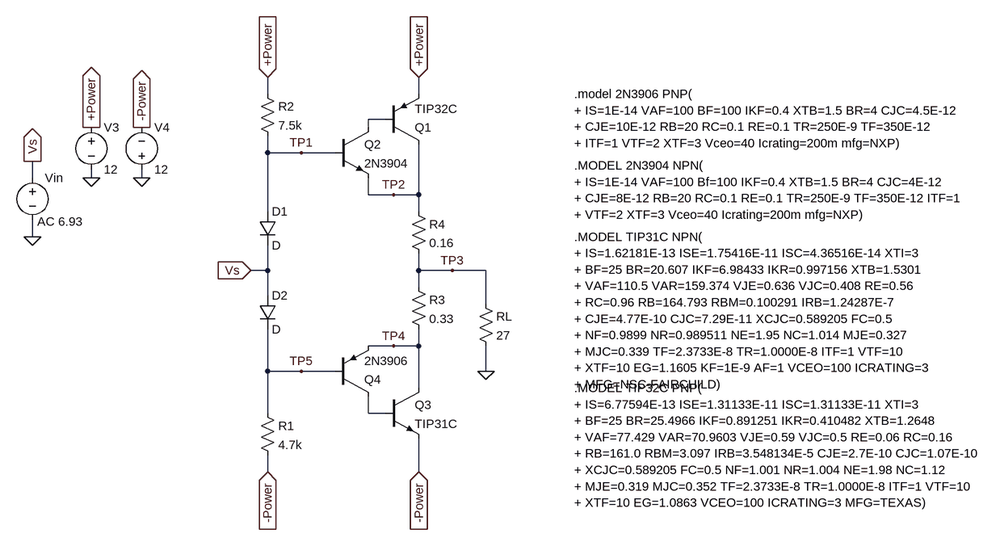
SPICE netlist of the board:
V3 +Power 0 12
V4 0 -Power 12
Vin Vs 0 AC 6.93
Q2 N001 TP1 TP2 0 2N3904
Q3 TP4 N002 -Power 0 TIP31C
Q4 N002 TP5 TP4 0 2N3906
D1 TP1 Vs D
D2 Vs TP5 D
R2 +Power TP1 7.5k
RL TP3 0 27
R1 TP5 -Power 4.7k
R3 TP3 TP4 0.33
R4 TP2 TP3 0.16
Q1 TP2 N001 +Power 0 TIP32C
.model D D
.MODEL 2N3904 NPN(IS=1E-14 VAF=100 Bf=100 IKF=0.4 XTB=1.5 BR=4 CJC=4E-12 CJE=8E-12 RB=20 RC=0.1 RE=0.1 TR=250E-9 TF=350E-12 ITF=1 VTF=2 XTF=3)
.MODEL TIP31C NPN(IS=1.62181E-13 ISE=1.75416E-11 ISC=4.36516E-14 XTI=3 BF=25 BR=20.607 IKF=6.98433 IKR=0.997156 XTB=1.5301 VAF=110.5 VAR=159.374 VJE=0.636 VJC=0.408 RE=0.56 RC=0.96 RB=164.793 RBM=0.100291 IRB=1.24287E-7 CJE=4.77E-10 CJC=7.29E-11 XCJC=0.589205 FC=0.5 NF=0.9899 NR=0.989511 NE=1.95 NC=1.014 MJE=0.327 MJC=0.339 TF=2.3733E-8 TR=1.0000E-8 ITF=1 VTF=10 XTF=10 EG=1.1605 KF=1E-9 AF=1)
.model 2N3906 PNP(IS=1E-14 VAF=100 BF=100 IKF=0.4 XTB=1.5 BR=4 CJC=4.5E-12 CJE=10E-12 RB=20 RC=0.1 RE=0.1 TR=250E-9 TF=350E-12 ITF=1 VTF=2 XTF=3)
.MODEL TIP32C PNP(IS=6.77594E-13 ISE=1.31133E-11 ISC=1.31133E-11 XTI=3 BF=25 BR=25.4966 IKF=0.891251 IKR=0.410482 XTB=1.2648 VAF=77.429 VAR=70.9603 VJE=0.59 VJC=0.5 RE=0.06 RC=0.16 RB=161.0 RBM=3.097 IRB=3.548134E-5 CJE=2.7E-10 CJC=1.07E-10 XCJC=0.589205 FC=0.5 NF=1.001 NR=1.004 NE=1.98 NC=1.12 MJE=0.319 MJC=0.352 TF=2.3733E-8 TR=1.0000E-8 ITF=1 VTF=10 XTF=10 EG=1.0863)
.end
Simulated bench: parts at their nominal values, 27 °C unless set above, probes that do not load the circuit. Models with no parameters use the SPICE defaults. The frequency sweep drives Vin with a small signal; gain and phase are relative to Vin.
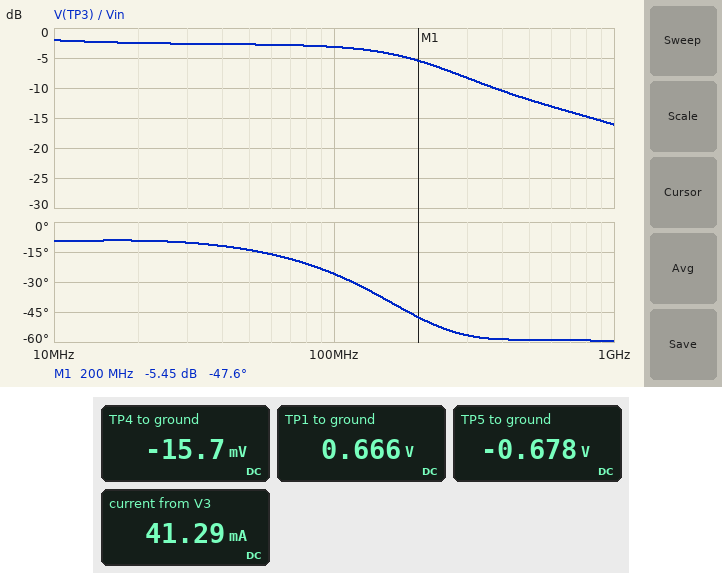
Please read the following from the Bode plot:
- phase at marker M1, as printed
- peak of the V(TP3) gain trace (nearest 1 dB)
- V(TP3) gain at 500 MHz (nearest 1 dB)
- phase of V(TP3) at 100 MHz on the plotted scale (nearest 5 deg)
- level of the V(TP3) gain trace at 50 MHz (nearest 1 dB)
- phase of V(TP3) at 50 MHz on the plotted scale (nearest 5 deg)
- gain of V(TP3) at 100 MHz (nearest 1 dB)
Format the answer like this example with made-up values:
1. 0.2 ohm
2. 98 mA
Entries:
1. -47.6 deg
2. -2 dB
3. -12 dB
4. -25 deg
5. -3 dB
6. -15 deg
7. -3 dB
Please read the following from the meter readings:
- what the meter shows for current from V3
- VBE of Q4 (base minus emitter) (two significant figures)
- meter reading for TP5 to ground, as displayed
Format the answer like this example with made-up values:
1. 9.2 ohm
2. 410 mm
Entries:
1. 41.29 mA
2. -660 mV
3. -0.678 V
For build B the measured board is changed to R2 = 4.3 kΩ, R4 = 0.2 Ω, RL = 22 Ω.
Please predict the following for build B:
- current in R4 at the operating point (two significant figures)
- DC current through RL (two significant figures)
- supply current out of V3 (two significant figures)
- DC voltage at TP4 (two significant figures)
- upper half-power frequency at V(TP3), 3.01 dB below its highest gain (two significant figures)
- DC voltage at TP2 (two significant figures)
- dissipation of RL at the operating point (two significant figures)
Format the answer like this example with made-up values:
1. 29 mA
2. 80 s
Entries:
1. 47 mA
2. 190 µA
3. 50 mA
4. -11 mV
5. 110 MHz
6. 14 mV
7. 790 nW
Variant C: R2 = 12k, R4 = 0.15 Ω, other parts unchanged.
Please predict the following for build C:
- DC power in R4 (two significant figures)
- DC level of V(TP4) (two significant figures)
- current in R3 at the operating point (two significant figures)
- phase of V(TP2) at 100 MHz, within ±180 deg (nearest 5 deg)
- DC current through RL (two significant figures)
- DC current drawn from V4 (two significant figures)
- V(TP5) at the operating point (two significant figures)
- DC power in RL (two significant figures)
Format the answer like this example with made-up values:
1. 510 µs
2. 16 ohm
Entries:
1. 170 µW
2. -20 mV
3. 34 mA
4. -30 deg
5. 330 µA
6. 36 mA
7. -680 mV
8. 2.9 µW
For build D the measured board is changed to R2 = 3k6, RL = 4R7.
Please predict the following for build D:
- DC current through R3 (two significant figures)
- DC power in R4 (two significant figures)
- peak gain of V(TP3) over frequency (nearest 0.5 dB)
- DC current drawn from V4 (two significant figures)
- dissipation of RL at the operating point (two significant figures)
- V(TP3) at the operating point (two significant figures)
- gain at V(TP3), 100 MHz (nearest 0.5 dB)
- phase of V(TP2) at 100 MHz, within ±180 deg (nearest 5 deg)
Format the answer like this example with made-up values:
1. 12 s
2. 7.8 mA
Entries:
1. 50 mA
2. 430 µW
3. -0.5 dB
4. 53 mA
5. 11 µW
6. 7.2 mV
7. -9.5 dB
8. -25 deg
